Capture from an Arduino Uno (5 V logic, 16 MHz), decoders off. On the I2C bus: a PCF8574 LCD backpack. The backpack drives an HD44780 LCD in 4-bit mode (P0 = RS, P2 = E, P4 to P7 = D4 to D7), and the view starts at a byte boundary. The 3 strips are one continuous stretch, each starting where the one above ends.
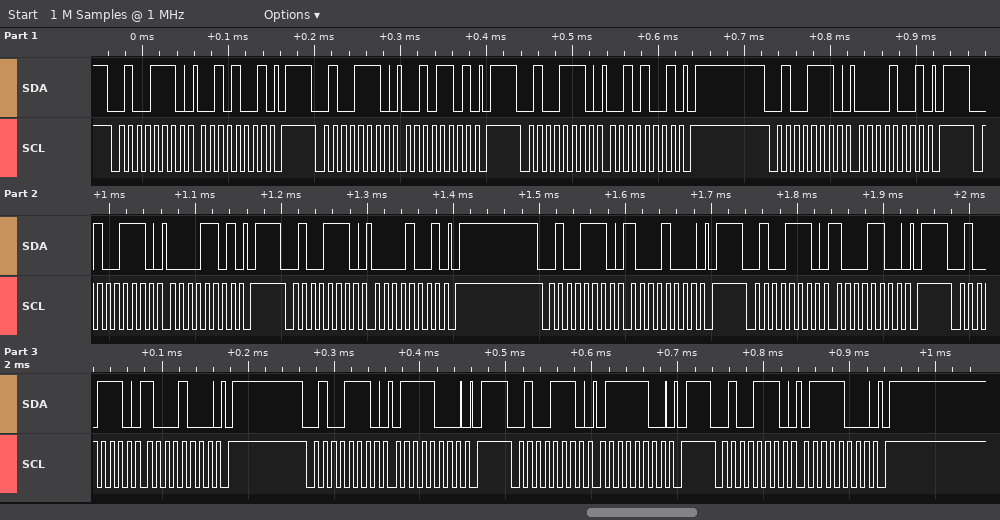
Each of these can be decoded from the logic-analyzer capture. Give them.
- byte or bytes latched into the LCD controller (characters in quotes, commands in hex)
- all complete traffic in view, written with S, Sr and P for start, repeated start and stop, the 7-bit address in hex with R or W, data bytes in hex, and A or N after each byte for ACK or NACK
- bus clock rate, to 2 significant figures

' ' 0x87
S 27W A 29 A P S 27W A 2D A P S 27W A 29 A P S 27W A 09 A P S 27W A 0D A P S 27W A 09 A P S 27W A 88 A P S 27W A 8C A P S 27W A 88 A P S 27W A 78 A P S 27W A 7C A P S 27W A 78 A P
100 kHz
